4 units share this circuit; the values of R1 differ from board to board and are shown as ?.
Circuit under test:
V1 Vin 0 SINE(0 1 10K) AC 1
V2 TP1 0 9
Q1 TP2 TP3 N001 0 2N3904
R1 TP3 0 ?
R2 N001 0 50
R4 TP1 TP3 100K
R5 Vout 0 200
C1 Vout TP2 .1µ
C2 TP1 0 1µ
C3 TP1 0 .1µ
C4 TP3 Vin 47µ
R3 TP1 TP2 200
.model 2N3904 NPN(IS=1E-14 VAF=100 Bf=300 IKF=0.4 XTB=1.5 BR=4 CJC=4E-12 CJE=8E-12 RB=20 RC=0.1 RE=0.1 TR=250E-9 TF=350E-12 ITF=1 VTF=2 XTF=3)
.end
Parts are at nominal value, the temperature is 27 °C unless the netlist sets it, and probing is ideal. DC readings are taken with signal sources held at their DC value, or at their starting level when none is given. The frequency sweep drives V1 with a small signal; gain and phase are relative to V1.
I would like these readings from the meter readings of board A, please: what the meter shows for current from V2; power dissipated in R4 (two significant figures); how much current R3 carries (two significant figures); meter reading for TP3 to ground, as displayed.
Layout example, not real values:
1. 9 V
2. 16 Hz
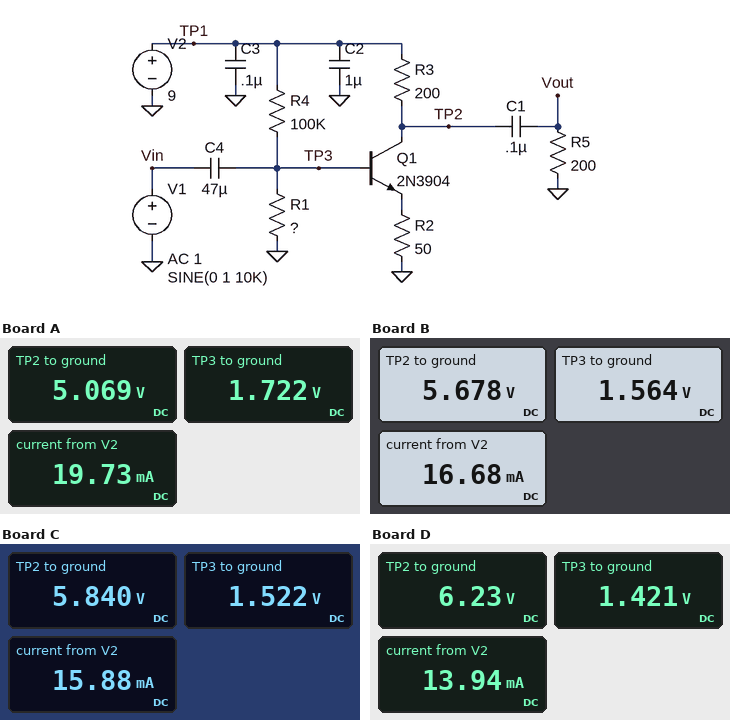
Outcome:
1. 19.73 mA
2. 530 µW
3. 20 mA
4. 1.722 V
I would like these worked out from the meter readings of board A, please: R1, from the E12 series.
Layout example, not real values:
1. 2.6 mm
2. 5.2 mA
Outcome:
1. 270 kΩ
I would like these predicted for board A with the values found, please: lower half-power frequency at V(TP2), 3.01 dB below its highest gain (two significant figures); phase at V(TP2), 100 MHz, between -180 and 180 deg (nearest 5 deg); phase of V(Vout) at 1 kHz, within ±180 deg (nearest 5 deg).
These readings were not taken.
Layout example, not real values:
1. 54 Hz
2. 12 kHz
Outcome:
1. 290 mHz
2. 145 deg
3. -105 deg
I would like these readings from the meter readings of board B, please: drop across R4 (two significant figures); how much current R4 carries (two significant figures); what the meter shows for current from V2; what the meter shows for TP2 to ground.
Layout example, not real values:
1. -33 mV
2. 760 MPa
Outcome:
1. 7.4 V
2. 74 µA
3. 16.68 mA
4. 5.678 V
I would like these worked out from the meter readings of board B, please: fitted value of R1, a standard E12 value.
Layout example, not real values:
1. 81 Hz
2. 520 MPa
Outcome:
1. 82 kΩ
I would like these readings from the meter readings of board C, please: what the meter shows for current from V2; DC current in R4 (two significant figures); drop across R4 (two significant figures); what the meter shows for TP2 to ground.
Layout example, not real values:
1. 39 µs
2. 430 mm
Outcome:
1. 15.88 mA
2. 75 µA
3. 7.5 V
4. 5.840 V
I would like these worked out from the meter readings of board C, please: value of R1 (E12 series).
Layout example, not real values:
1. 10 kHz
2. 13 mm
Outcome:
1. 68 kΩ
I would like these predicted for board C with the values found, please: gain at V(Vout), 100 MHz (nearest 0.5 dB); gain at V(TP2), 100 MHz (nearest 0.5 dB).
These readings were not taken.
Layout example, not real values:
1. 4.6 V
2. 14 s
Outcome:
1. 5.0 dB
2. 5.0 dB
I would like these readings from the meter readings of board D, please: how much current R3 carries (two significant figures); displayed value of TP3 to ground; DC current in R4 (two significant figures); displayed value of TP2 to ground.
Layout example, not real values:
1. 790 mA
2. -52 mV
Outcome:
1. 14 mA
2. 1.421 V
3. 76 µA
4. 6.23 V
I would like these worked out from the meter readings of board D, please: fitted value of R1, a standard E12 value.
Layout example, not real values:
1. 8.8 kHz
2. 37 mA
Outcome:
1. 47 kΩ
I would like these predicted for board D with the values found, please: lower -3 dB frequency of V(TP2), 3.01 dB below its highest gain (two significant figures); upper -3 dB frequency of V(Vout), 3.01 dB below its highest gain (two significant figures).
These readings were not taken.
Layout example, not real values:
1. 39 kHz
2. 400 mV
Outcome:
1. 330 mHz
2. 290 MHz
